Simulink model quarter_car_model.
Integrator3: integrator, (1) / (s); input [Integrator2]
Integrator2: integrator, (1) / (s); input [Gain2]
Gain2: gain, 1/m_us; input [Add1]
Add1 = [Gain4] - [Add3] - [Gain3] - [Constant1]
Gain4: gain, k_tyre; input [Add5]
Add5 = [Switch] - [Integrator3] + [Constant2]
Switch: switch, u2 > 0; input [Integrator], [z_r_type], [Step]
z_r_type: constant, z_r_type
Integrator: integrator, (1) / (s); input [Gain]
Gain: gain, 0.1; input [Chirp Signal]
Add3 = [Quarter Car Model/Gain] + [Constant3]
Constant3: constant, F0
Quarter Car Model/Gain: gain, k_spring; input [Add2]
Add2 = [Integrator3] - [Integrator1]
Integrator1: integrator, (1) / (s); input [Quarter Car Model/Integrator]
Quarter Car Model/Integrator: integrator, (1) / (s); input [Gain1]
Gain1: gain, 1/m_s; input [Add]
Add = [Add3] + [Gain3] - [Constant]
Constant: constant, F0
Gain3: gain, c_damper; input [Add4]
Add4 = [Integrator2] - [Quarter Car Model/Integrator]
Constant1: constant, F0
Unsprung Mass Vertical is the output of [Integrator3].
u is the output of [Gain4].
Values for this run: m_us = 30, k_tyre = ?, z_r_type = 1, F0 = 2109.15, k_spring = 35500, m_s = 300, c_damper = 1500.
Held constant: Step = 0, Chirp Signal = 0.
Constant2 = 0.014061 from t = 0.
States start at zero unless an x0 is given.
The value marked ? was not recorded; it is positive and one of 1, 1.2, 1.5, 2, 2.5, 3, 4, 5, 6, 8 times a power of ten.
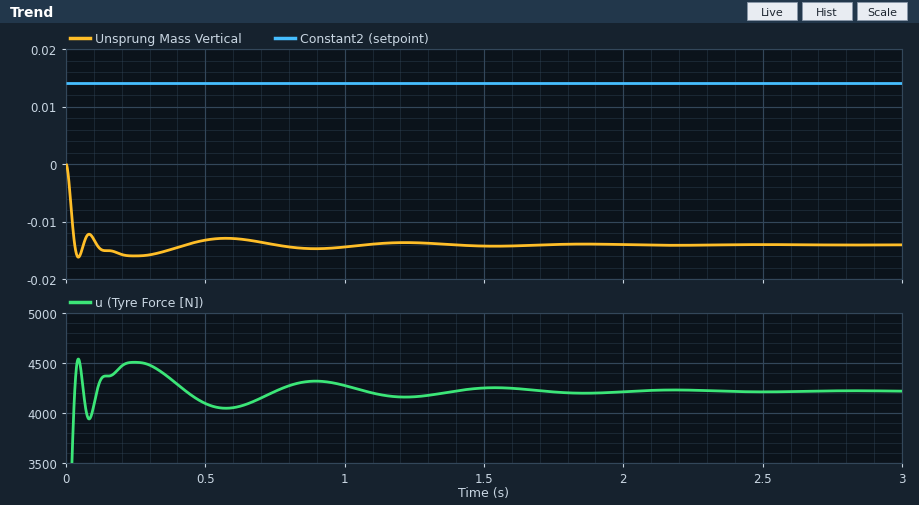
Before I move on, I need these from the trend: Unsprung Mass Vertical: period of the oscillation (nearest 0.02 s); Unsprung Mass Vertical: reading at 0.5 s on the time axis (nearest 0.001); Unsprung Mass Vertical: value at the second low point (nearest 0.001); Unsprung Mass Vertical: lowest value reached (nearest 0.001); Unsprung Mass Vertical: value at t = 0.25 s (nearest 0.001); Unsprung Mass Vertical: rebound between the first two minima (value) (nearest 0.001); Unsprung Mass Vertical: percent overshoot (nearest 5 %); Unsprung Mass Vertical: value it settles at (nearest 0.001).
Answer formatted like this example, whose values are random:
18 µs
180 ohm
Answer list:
0.20 s
-0.013
-0.016
-0.016
-0.016
-0.012
15 %
-0.014
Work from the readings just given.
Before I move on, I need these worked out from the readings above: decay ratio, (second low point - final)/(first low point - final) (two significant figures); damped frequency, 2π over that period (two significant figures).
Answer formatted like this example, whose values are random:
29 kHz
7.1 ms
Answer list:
1.0
31 rad/s
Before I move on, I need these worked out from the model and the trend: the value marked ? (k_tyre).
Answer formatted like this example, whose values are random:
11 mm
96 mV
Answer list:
150000
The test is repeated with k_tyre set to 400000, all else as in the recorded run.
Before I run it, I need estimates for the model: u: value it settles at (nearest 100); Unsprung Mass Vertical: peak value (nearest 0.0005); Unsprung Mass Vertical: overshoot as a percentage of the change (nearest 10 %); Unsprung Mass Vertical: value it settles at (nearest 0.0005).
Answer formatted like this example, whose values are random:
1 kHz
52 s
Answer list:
4200
0.0050
40 %
0.0035
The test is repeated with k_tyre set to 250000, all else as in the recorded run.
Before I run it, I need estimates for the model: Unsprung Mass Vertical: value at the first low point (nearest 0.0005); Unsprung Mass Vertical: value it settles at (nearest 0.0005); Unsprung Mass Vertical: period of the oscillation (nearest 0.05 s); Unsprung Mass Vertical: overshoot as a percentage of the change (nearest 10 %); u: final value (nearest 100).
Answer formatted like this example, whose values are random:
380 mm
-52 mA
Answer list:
-0.0035
-0.0030
0.20 s
30 %
4200
